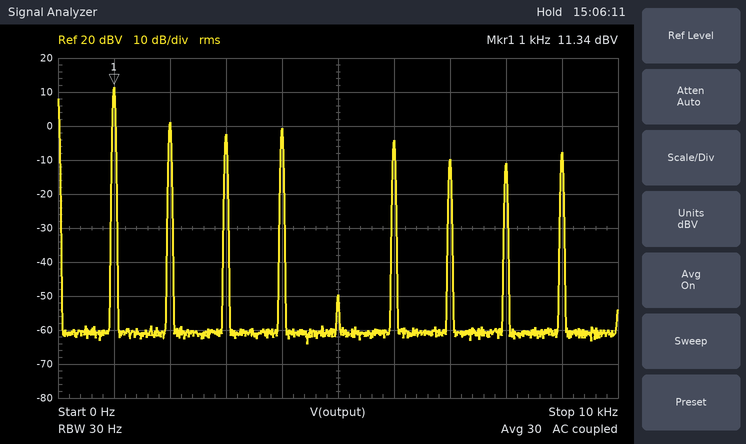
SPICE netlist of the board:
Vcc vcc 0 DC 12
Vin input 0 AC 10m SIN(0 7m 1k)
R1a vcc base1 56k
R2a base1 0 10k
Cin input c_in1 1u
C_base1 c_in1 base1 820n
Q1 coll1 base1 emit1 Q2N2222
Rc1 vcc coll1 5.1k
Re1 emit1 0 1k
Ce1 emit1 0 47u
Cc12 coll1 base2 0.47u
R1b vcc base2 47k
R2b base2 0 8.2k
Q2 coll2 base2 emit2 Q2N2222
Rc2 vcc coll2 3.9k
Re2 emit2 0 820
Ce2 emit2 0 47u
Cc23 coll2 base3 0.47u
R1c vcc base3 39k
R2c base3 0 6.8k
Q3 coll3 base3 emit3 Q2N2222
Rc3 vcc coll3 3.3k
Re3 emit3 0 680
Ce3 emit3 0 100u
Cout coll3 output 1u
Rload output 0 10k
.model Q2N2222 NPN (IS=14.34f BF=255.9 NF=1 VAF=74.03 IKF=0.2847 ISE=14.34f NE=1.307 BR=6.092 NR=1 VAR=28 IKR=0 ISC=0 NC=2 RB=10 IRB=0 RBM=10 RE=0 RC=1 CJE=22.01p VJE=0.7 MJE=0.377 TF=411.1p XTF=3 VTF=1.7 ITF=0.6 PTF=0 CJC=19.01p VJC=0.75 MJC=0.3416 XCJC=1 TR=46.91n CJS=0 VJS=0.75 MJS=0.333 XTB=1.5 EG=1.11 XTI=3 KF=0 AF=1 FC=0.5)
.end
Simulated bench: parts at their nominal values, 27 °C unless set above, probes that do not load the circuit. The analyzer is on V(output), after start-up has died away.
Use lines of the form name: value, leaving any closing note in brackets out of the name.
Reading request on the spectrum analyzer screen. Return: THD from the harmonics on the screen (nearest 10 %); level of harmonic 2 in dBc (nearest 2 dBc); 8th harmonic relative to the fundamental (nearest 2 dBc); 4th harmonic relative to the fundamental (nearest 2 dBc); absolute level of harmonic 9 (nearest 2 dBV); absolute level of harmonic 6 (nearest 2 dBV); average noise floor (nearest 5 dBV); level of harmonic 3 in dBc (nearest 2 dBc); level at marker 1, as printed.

THD from the harmonics on the screen: 50 %
level of harmonic 2 in dBc: -10 dBc
8th harmonic relative to the fundamental: -22 dBc
4th harmonic relative to the fundamental: -12 dBc
absolute level of harmonic 9: -8 dBV
absolute level of harmonic 6: -4 dBV
average noise floor: -60 dBV
level of harmonic 3 in dBc: -14 dBc
level at marker 1, as printed: 11.34 dBV
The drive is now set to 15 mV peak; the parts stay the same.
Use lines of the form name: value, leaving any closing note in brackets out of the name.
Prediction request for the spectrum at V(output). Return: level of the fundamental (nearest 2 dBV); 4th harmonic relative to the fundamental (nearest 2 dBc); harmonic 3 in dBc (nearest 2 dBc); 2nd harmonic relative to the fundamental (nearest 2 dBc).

level of the fundamental: 12 dBV
4th harmonic relative to the fundamental: -14 dBc
harmonic 3 in dBc: -12 dBc
2nd harmonic relative to the fundamental: -12 dBc
